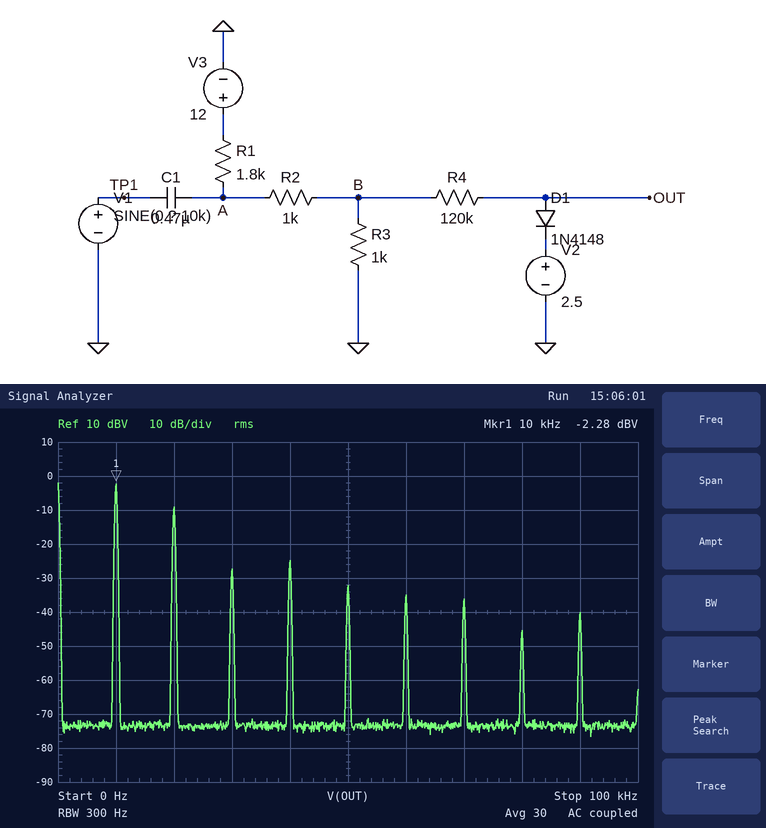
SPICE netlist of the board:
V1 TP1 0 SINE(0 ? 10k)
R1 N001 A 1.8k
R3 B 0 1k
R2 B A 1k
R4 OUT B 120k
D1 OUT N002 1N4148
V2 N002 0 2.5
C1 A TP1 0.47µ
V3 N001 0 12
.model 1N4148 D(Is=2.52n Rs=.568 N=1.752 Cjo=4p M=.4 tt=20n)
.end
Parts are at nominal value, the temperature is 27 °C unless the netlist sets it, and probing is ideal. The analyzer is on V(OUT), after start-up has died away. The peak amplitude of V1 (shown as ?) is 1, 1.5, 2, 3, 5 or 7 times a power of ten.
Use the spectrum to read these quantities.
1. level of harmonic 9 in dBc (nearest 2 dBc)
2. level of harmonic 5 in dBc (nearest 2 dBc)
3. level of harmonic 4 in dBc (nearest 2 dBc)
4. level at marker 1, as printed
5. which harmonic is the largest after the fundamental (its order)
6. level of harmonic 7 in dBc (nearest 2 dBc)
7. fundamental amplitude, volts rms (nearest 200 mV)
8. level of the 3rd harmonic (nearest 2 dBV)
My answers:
-38 dBc
-30 dBc
-22 dBc
-2.28 dBV
2
-34 dBc
800 mV
-28 dBV
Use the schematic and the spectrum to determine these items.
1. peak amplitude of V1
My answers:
5 V
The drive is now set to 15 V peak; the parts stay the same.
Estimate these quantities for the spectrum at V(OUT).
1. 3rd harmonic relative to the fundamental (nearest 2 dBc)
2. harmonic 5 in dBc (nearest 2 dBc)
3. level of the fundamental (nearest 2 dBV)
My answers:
-36 dBc
-40 dBc
8 dBV
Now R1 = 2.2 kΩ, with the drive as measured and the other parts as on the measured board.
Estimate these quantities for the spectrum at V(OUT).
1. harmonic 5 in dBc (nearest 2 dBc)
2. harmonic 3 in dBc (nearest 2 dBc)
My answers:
-48 dBc
-48 dBc
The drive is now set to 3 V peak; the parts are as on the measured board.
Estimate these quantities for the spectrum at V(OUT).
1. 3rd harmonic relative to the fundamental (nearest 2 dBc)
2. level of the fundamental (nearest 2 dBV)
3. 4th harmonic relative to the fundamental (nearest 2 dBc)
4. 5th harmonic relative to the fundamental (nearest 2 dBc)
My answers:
-20 dBc
-8 dBV
-26 dBc
-26 dBc
